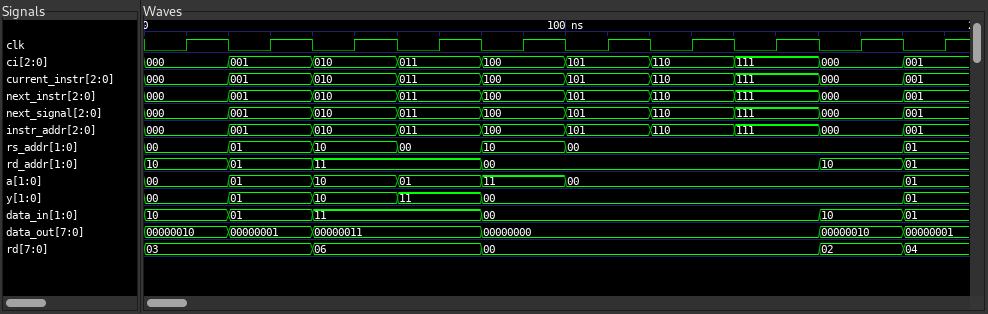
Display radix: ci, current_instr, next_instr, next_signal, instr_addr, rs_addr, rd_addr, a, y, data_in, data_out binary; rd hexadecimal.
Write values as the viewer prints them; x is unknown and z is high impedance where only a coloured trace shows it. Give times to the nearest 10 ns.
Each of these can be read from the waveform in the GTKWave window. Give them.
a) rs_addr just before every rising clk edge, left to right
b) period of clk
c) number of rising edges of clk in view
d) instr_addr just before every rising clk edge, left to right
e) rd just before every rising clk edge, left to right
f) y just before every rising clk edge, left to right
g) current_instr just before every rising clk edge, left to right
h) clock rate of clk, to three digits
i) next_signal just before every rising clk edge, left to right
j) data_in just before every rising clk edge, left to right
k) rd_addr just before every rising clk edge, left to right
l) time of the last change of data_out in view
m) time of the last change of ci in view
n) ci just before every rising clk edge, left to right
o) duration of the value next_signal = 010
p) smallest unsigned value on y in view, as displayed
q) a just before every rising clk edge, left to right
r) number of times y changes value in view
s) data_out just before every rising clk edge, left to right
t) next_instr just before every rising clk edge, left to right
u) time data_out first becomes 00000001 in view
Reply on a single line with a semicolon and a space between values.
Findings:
00, 01, 10, 00, 10, 00, 00, 00, 00, 01; 20 ns; 10; 000, 001, 010, 011, 100, 101, 110, 111, 000, 001; 03, 03, 06, 06, 00, 00, 00, 00, 02, 04; 00, 01, 10, 11, 00, 00, 00, 00, 00, 01; 000, 001, 010, 011, 100, 101, 110, 111, 000, 001; 50.0 MHz; 000, 001, 010, 011, 100, 101, 110, 111, 000, 001; 10, 01, 11, 11, 00, 00, 00, 00, 10, 01; 10, 01, 11, 11, 00, 00, 00, 00, 10, 01; 180 ns; 180 ns; 000, 001, 010, 011, 100, 101, 110, 111, 000, 001; 20 ns; 00; 00, 01, 10, 01, 11, 00, 00, 00, 00, 01; 5; 00000010, 00000001, 00000011, 00000011, 00000000, 00000000, 00000000, 00000000, 00000010, 00000001; 000, 001, 010, 011, 100, 101, 110, 111, 000, 001; 20 ns
